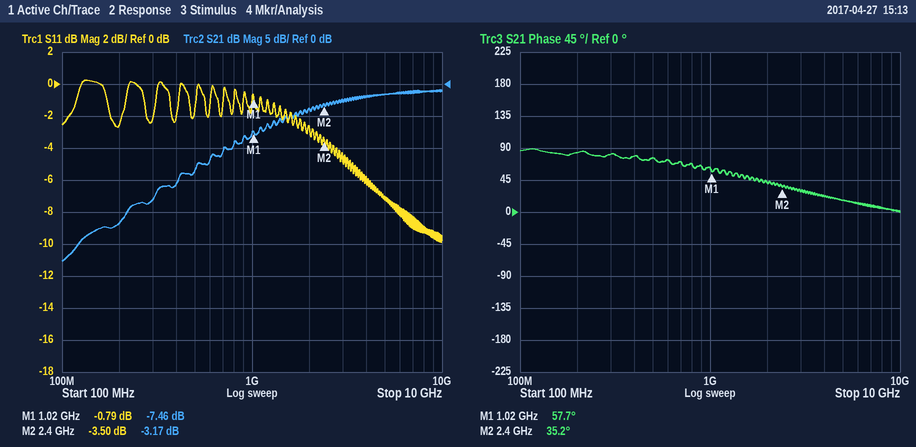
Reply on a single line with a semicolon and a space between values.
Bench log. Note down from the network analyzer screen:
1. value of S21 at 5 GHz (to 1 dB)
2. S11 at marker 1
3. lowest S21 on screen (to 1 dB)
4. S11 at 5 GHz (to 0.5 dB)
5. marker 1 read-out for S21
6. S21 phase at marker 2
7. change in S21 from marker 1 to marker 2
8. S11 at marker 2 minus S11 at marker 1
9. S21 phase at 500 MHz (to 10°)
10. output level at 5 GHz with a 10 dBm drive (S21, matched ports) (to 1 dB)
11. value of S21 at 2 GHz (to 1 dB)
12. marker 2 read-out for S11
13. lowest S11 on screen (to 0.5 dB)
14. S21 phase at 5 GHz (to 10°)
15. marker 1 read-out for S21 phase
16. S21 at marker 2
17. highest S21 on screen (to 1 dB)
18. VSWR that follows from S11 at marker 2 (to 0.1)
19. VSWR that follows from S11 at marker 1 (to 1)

-2 dB; -0.79 dB; -28 dB; -7.0 dB; -7.46 dB; 35.2°; 4.29 dB; -2.71 dB; 80°; 8 dBm; -4 dB; -3.50 dB; -10.0 dB; 20°; 57.7°; -3.17 dB; -1 dB; 5.0; 22
